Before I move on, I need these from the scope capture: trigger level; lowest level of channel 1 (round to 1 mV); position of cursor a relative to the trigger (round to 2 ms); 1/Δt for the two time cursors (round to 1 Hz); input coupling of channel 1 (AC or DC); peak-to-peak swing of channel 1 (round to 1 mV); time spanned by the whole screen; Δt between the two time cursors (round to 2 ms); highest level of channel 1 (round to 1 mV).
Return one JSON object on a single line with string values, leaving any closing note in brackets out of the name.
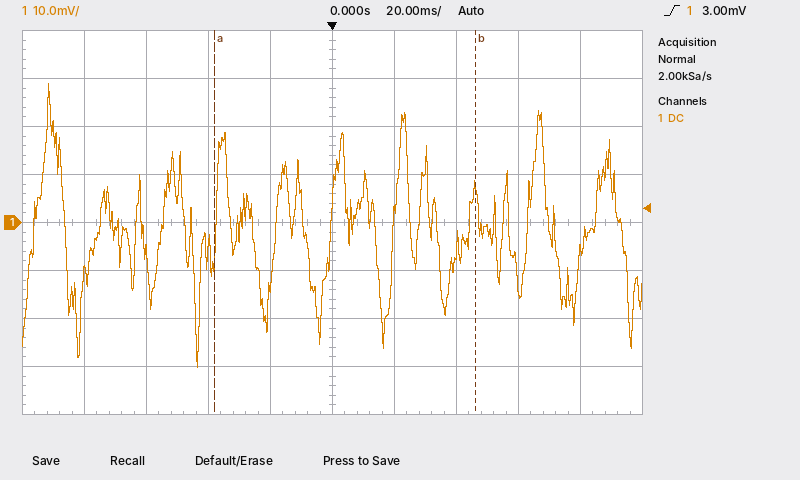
{"trigger level": "3.00 mV", "lowest level of channel 1": "-30 mV", "position of cursor a relative to the trigger": "-38 ms", "1/Δt for the two time cursors": "12 Hz", "input coupling of channel 1": "DC", "peak-to-peak swing of channel 1": "59 mV", "time spanned by the whole screen": "200 ms", "Δt between the two time cursors": "84 ms", "highest level of channel 1": "29 mV"}
